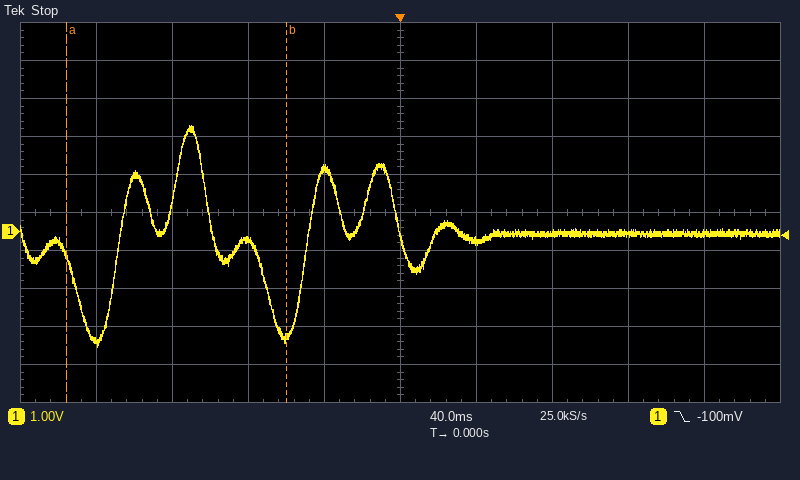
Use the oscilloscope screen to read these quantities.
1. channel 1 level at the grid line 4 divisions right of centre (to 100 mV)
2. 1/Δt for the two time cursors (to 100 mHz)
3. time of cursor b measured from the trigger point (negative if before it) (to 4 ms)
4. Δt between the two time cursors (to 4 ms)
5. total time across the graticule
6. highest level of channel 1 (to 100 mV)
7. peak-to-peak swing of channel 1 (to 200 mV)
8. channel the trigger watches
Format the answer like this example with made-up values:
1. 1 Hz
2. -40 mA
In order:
1. -100 mV
2. 8.6 Hz
3. -60 ms
4. 116 ms
5. 400 ms
6. 2.8 V
7. 5.8 V
8. channel 1
